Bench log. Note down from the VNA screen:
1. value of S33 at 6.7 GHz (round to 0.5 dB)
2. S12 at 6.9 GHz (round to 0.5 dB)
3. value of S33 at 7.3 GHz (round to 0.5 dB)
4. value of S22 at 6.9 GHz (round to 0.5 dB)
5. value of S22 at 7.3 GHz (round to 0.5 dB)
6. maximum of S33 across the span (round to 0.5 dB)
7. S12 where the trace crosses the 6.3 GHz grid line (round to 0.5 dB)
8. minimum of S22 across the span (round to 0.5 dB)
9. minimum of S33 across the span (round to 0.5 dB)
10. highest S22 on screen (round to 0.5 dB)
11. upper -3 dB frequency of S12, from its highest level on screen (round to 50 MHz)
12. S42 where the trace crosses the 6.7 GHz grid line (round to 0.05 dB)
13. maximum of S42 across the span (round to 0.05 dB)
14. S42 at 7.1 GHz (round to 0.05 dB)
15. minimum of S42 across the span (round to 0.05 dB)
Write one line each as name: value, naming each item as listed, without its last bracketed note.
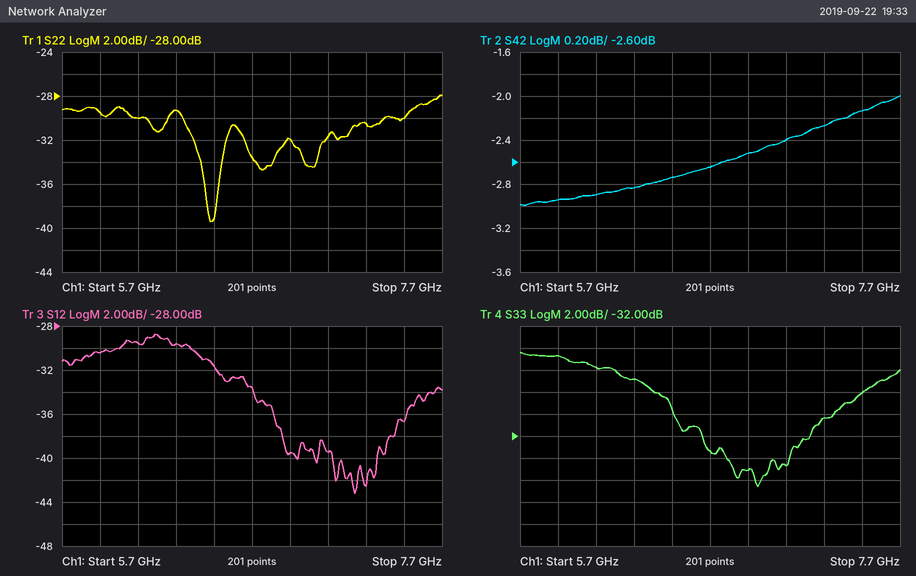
value of S33 at 6.7 GHz: -33.5 dB
S12 at 6.9 GHz: -39.5 dB
value of S33 at 7.3 GHz: -30.5 dB
value of S22 at 6.9 GHz: -32.0 dB
value of S22 at 7.3 GHz: -30.5 dB
maximum of S33 across the span: -24.5 dB
S12 where the trace crosses the 6.3 GHz grid line: -29.5 dB
minimum of S22 across the span: -39.5 dB
minimum of S33 across the span: -36.5 dB
highest S22 on screen: -28.0 dB
upper -3 dB frequency of S12, from its highest level on screen: 6.50 GHz
S42 where the trace crosses the 6.7 GHz grid line: -2.65 dB
maximum of S42 across the span: -2.00 dB
S42 at 7.1 GHz: -2.40 dB
minimum of S42 across the span: -3.00 dB
